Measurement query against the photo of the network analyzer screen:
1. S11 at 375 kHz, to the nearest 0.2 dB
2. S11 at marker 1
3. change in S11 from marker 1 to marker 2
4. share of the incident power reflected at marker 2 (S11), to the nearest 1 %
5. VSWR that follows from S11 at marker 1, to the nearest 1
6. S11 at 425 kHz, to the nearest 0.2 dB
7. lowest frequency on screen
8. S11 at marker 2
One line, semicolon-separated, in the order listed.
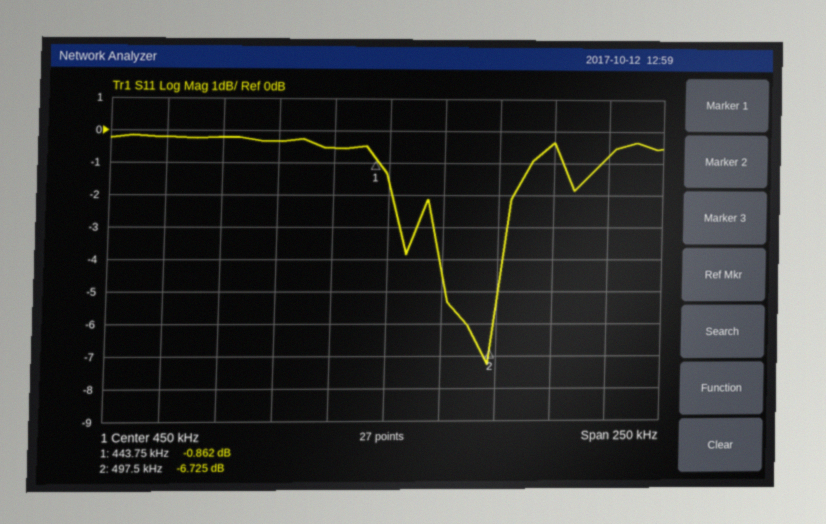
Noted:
-0.2 dB; -0.862 dB; -5.863 dB; 21 %; 20; -0.6 dB; 325 kHz; -6.725 dB
